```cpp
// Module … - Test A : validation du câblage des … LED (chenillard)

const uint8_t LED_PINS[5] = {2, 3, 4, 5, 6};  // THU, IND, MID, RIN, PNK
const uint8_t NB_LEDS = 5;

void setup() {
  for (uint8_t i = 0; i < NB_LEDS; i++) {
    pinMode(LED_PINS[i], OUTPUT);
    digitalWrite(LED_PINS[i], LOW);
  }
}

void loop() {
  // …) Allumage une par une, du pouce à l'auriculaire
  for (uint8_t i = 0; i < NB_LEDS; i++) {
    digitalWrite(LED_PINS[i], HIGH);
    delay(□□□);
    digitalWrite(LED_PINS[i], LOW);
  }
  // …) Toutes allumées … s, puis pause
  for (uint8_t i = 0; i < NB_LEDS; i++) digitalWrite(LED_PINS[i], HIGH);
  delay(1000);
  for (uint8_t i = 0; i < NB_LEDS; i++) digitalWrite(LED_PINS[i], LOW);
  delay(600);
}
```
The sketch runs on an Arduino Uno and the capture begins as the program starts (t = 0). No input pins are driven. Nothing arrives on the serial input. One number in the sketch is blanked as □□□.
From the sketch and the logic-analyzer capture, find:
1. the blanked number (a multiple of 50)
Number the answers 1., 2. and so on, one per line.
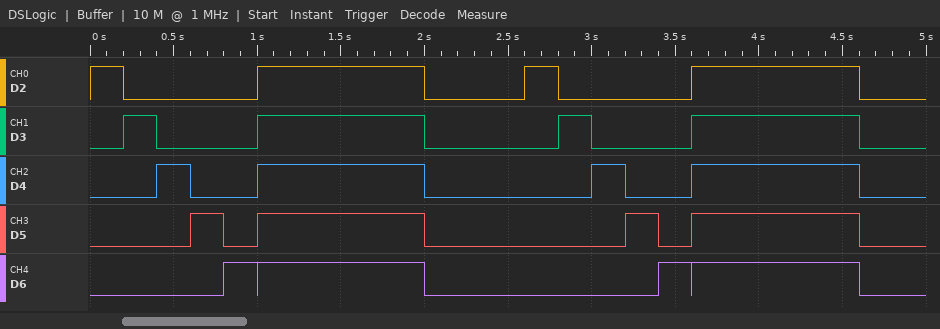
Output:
1. 200
